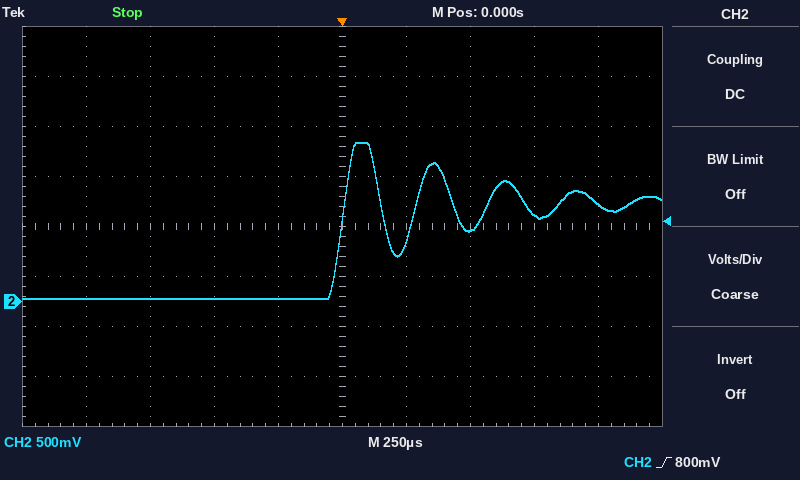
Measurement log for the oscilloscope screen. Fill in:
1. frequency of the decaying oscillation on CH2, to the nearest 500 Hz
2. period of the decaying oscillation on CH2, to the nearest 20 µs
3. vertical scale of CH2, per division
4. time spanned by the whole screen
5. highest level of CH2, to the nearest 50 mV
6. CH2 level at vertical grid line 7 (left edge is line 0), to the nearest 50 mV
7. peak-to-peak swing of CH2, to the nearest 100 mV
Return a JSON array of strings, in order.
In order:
["3.5 kHz", "280 µs", "500 mV", "2.5 ms", "1.60 V", "700 mV", "1.60 V"]
